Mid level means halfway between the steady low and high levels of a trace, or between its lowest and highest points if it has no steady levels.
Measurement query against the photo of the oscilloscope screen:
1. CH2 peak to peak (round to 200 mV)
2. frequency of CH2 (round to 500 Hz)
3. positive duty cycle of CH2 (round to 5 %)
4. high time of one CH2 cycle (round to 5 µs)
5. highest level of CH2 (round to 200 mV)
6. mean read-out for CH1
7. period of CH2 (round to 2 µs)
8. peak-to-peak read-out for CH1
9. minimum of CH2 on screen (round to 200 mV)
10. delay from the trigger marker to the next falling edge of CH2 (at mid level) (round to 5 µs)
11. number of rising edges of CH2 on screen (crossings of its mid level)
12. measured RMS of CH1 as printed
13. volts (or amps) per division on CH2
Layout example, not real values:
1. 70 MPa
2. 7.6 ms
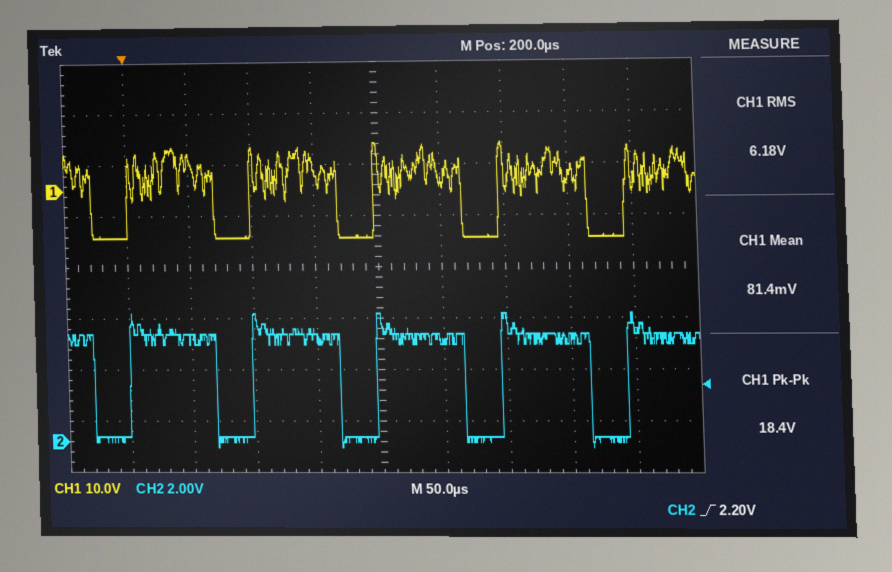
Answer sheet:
1. 5.2 V
2. 10.0 kHz
3. 70 %
4. 70 µs
5. 5.0 V
6. 81.4 mV
7. 98 µs
8. 18.4 V
9. -200 mV
10. 70 µs
11. 5
12. 6.18 V
13. 2 V
